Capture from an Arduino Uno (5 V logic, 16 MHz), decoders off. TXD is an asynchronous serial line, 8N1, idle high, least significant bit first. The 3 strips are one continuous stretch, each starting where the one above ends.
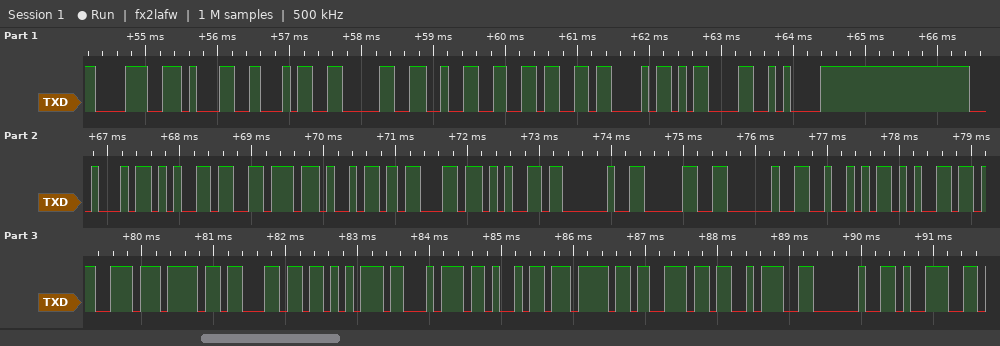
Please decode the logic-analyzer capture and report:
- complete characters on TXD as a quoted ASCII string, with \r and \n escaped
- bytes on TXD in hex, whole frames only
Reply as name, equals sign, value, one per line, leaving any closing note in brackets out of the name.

complete characters on TXD as a quoted ASCII string, with \r and \n escaped = "814026C\r\nDevice 0 Resolution: 9"
bytes on TXD in hex, whole frames only = 38 31 34 30 32 36 43 0D 0A 44 65 76 69 63 65 20 30 20 52 65 73 6F 6C 75 74 69 6F 6E 3A 20 39
